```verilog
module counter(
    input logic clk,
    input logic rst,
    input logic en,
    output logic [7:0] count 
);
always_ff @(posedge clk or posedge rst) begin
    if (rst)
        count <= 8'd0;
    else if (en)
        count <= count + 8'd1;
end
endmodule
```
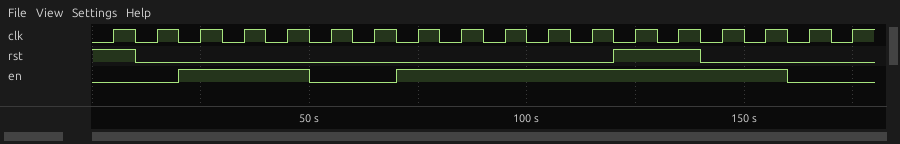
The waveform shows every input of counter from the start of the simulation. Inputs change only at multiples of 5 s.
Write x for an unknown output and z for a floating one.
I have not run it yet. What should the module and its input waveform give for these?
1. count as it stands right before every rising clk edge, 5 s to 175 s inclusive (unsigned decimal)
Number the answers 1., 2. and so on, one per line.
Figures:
1. 0, 0, 0, 1, 2, 3, 3, 3, 4, 5, 6, 7, 0, 0, 0, 1, 2, 2
